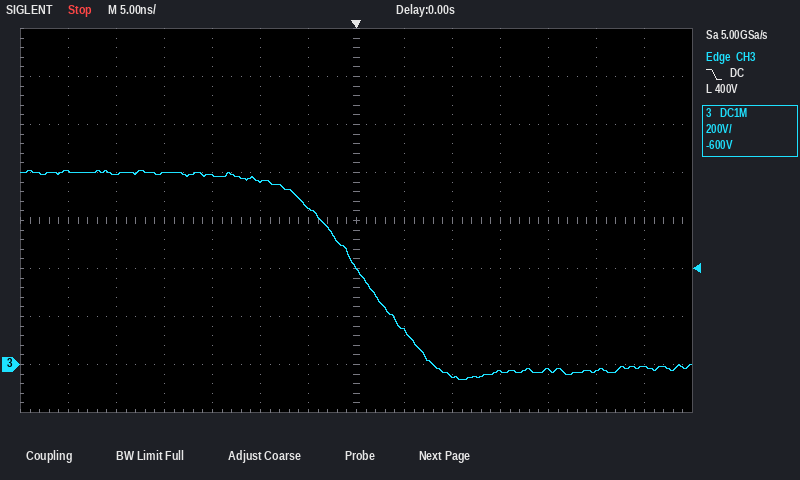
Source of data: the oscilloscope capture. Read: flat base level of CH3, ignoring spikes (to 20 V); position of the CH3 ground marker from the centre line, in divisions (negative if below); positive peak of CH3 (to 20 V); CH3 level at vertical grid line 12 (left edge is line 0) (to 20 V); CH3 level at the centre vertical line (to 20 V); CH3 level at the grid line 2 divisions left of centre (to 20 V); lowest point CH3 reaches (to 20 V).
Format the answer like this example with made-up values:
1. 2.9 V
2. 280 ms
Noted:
1. -20 V
2. -3.0 div
3. 800 V
4. -20 V
5. 400 V
6. 760 V
7. -60 V
